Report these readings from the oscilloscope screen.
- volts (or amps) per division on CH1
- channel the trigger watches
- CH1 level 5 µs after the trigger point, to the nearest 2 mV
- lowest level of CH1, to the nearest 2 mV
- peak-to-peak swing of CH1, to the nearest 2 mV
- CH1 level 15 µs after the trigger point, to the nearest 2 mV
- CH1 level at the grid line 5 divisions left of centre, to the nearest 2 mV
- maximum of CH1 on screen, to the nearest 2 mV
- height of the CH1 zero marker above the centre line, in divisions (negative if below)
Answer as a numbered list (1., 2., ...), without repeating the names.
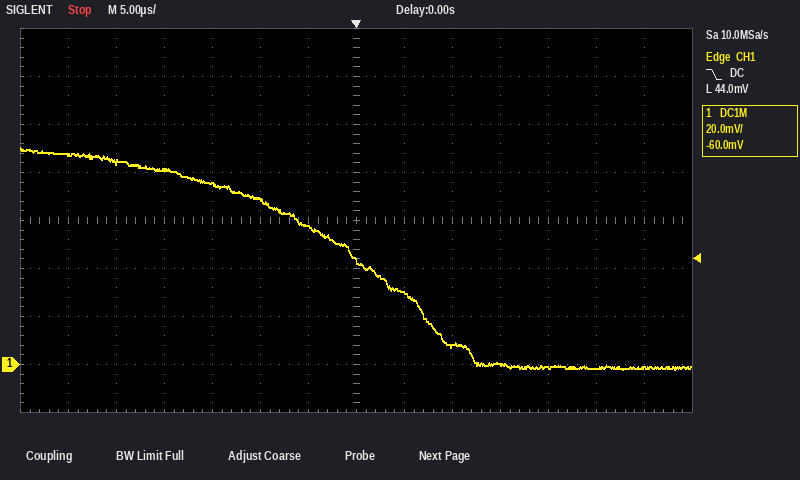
1. 20 mV
2. CH1
3. 30 mV
4. -2 mV
5. 92 mV
6. 0 mV
7. 84 mV
8. 90 mV
9. -3.0 div
